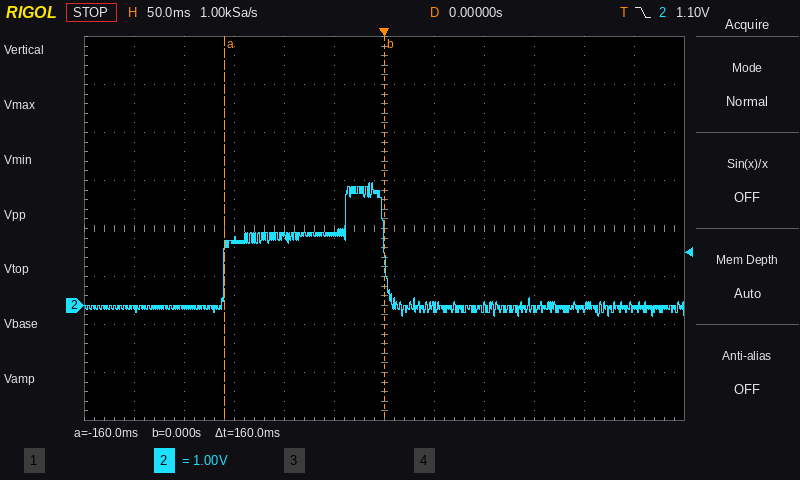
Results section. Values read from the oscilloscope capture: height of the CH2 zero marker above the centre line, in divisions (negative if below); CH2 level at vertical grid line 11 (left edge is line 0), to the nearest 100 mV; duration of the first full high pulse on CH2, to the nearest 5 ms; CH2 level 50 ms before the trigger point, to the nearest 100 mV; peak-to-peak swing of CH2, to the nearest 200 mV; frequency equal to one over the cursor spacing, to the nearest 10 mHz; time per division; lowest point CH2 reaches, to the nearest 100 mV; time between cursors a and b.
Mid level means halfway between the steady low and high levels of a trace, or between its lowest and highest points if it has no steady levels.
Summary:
-1.6 div
-100 mV
160 ms
1.5 V
2.8 V
6.25 Hz
50 ms
-200 mV
160 ms
